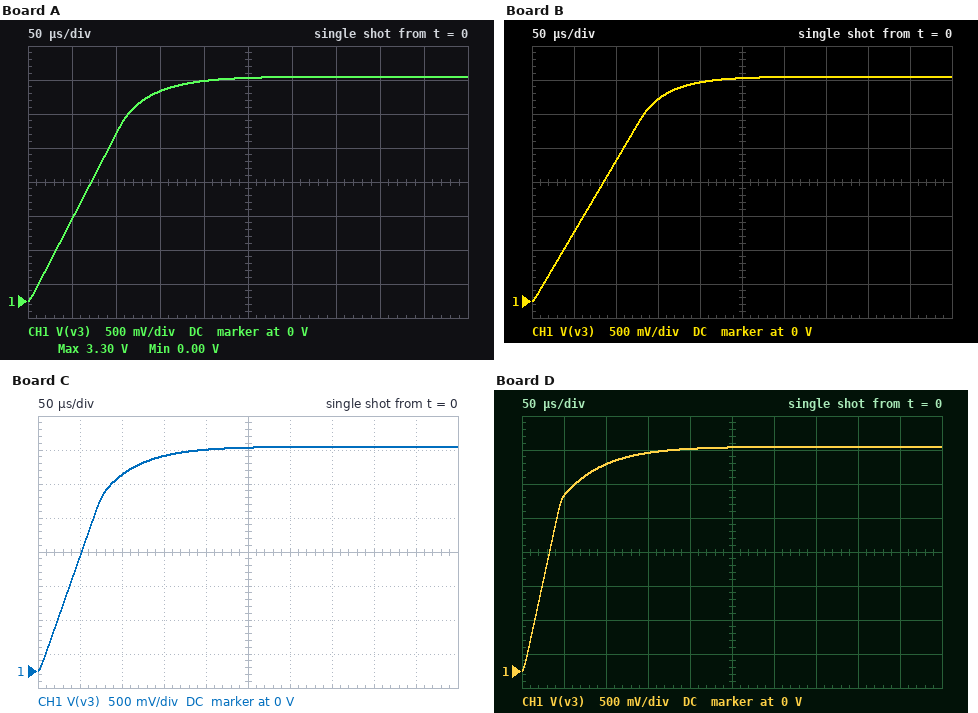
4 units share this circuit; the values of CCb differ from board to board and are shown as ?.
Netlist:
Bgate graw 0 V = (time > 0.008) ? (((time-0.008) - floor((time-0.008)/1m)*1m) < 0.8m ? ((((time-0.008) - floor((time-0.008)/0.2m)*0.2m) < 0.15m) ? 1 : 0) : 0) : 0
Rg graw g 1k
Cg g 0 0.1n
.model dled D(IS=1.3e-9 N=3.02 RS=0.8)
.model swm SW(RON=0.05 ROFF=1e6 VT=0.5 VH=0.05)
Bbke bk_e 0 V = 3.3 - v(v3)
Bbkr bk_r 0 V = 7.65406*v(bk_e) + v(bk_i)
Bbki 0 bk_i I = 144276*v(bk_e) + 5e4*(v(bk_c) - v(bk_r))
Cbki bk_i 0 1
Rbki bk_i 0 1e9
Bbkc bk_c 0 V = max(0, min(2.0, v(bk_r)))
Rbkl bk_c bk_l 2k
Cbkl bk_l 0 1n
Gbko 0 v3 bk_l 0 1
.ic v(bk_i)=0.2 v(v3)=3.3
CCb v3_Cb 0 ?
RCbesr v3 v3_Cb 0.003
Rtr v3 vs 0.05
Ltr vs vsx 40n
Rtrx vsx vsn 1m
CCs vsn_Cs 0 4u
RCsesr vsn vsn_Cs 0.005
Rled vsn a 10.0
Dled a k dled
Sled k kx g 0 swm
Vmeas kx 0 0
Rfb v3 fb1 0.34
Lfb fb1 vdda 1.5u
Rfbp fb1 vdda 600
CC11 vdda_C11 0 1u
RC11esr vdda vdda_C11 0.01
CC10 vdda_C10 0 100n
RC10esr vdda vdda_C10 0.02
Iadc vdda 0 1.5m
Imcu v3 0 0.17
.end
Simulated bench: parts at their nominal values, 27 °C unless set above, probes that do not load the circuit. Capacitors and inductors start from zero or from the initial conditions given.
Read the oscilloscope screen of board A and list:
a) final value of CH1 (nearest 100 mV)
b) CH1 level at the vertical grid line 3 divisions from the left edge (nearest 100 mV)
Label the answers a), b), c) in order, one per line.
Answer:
a) 3.3 V
b) 3.1 V
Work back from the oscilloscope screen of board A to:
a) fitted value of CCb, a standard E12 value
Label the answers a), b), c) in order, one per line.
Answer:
a) 68 µF
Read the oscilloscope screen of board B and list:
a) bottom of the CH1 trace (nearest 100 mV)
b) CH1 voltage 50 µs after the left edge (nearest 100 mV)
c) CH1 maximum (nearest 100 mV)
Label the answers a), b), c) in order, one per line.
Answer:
a) 0 V
b) 1.0 V
c) 3.3 V
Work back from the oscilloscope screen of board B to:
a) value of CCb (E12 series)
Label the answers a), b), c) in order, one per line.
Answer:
a) 82 µF
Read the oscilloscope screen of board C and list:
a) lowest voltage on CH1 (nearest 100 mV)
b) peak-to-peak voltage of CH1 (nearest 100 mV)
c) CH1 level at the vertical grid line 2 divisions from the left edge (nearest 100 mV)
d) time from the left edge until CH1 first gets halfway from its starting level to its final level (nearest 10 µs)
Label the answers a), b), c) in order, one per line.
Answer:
a) 0 V
b) 3.3 V
c) 2.9 V
d) 50 µs
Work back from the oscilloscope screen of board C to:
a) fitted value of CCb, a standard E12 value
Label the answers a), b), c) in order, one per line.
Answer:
a) 47 µF
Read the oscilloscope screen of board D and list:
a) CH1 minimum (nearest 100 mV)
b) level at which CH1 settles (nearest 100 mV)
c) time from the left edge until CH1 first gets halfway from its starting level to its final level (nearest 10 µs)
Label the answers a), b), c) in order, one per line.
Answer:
a) 0 V
b) 3.3 V
c) 30 µs
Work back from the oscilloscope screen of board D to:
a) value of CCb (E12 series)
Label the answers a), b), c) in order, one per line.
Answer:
a) 27 µF
